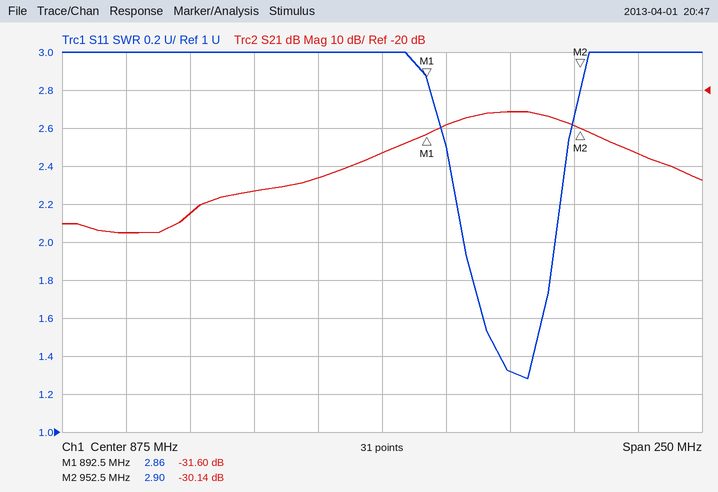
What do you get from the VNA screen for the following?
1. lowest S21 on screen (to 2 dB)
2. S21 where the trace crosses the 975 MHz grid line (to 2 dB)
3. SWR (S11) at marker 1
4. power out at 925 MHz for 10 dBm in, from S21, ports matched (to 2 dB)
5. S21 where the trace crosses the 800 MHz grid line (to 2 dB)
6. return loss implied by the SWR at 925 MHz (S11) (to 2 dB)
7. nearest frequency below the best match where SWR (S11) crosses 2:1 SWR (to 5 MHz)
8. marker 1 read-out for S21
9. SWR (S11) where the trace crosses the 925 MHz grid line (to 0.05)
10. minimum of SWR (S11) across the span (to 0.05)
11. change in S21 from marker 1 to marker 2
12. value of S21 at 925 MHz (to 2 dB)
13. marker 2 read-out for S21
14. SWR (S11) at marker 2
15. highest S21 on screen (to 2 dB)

-58 dB
-36 dB
2.86
-16 dBm
-52 dB
18 dB
905 MHz
-31.60 dB
1.30
1.30
1.46 dB
-26 dB
-30.14 dB
2.90
-26 dB
